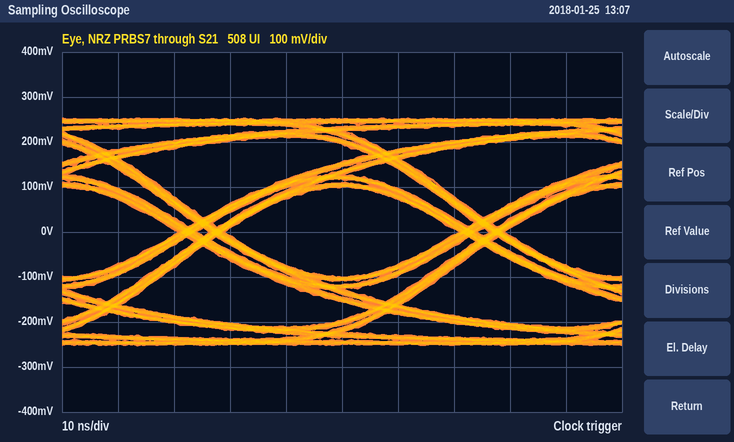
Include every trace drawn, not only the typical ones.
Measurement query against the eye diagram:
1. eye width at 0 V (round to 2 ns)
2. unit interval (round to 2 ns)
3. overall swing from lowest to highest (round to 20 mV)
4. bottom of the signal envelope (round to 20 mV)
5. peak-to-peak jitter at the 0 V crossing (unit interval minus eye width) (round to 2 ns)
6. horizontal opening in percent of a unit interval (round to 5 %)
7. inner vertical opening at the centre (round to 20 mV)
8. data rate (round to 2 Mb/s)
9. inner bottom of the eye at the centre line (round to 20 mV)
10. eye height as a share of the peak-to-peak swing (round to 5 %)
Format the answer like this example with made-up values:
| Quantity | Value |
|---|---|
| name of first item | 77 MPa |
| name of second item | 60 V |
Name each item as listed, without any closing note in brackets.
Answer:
| Quantity | Value |
|---|---|
| eye width at 0 V | 42 ns |
| unit interval | 50 ns |
| overall swing from lowest to highest | 500 mV |
| bottom of the signal envelope | -260 mV |
| peak-to-peak jitter at the 0 V crossing (unit interval minus eye width) | 8 ns |
| horizontal opening in percent of a unit interval | 85 % |
| inner vertical opening at the centre | 200 mV |
| data rate | 20 Mb/s |
| inner bottom of the eye at the centre line | -100 mV |
| eye height as a share of the peak-to-peak swing | 40 % |
